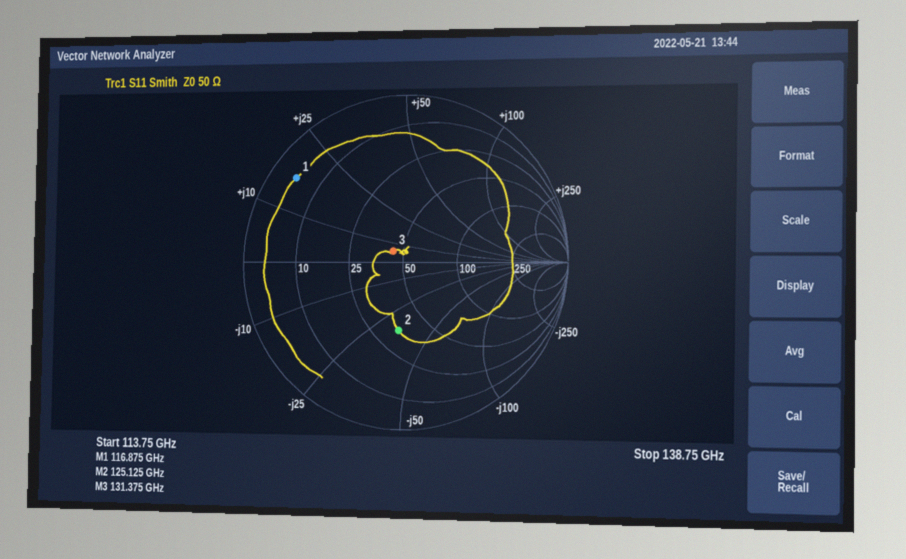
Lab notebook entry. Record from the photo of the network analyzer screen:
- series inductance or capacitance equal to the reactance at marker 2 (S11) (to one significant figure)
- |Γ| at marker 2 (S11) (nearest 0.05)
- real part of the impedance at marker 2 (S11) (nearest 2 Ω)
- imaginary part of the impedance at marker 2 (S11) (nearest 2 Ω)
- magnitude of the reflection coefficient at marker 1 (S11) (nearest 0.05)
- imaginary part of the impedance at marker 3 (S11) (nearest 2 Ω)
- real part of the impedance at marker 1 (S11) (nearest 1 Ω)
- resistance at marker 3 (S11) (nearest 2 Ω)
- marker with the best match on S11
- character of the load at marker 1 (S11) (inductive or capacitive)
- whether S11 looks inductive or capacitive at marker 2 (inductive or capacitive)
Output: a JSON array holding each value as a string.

["40 fF", "0.40", "34 Ω", "-34 Ω", "0.85", "+6 Ω", "5 Ω", "44 Ω", "marker 3", "inductive", "capacitive"]
